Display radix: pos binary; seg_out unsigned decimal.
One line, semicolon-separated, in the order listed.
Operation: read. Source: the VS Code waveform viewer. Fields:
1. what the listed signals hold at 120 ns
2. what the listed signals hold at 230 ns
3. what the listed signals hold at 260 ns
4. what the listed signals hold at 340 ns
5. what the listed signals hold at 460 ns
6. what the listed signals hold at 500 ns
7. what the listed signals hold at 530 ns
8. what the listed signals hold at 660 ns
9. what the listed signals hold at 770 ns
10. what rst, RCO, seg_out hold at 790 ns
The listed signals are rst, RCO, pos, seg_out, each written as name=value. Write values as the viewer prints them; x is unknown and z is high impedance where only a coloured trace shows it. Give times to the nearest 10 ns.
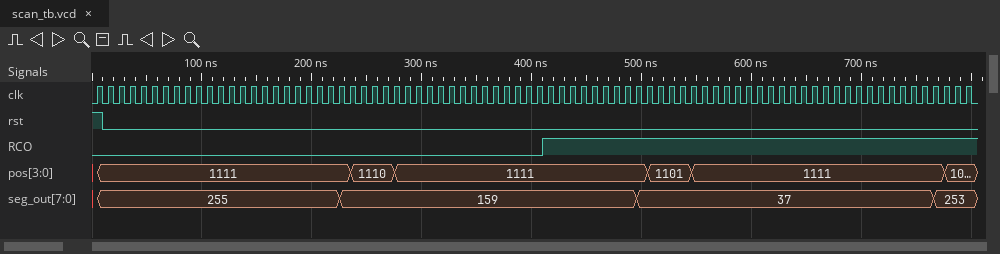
rst=0, RCO=0, pos=1111, seg_out=255; rst=0, RCO=0, pos=1111, seg_out=159; rst=0, RCO=0, pos=1110, seg_out=159; rst=0, RCO=0, pos=1111, seg_out=159; rst=0, RCO=1, pos=1111, seg_out=159; rst=0, RCO=1, pos=1111, seg_out=37; rst=0, RCO=1, pos=1101, seg_out=37; rst=0, RCO=1, pos=1111, seg_out=37; rst=0, RCO=1, pos=1111, seg_out=253; rst=0, RCO=1, seg_out=253
